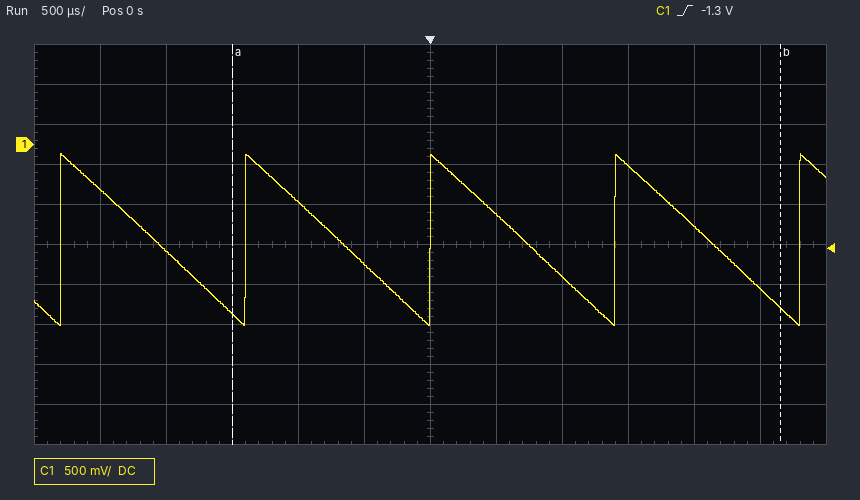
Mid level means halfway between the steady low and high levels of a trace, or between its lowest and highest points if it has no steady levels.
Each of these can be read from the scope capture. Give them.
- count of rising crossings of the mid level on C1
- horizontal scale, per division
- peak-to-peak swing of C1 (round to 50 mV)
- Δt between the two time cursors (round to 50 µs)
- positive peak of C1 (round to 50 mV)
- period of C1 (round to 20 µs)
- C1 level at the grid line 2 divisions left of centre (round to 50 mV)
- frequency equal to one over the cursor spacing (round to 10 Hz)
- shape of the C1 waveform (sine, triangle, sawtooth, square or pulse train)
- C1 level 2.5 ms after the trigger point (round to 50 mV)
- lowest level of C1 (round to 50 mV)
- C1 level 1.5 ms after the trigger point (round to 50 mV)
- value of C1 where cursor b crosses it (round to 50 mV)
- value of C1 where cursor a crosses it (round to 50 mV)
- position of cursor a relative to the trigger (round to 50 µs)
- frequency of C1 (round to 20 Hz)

5
500 µs
2.15 V
4.15 ms
-100 mV
1.40 ms
-700 mV
240 Hz
sawtooth
-1.80 V
-2.25 V
-250 mV
-2.05 V
-2.10 V
-1.50 ms
720 Hz
